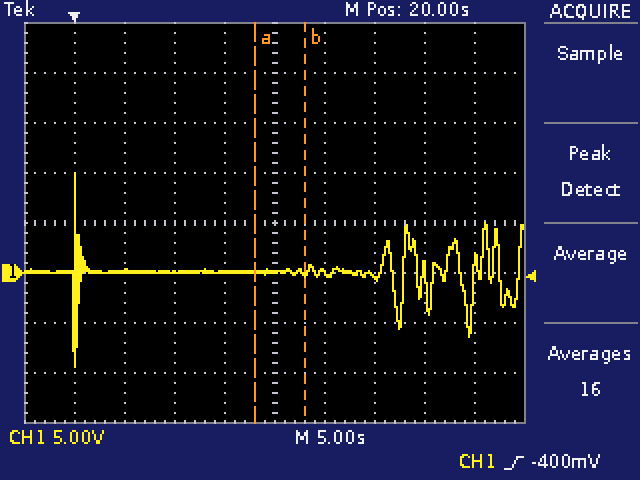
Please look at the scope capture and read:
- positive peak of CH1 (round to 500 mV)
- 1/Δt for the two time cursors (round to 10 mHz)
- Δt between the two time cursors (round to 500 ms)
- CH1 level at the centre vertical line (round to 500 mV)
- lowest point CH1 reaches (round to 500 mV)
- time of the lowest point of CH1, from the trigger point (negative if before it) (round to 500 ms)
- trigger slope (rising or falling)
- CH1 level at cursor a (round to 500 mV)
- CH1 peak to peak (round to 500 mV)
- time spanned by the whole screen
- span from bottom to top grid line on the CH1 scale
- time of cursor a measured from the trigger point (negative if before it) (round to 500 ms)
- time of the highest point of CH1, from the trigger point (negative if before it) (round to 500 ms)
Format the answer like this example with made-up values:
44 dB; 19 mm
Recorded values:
10.0 V; 200 mHz; 5.0 s; 0.0 V; -9.5 V; 0.0 s; rising; 0.0 V; 19.5 V; 50 s; 40 V; +18.0 s; 0.0 s
